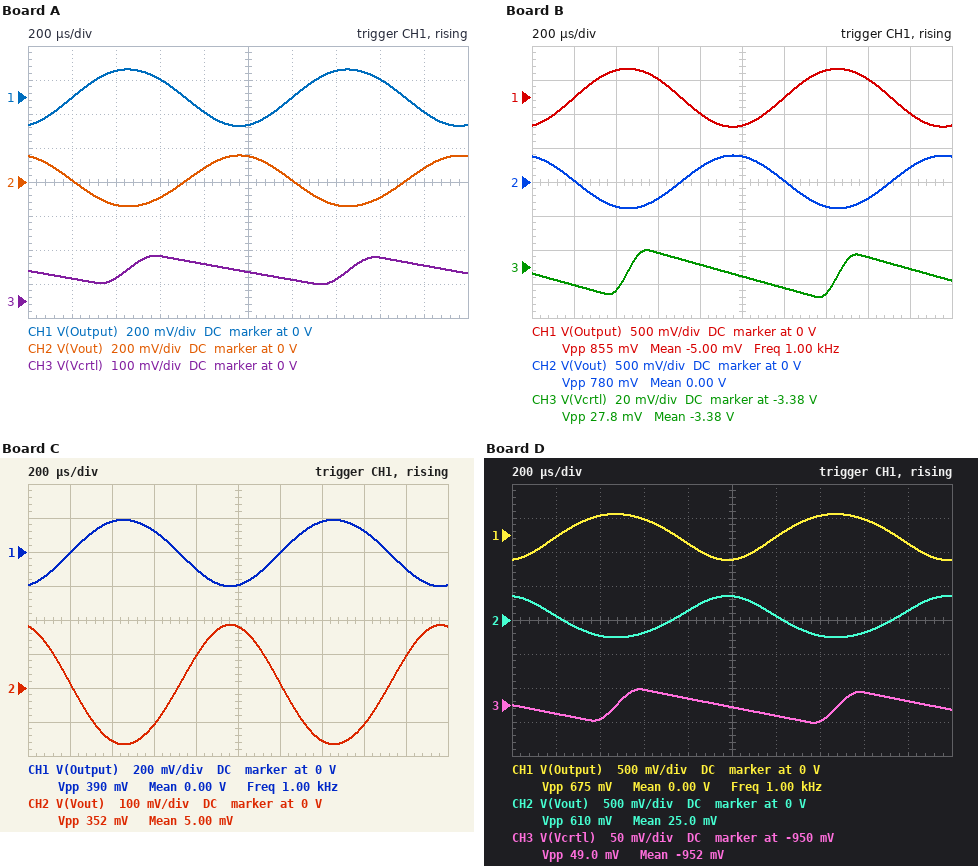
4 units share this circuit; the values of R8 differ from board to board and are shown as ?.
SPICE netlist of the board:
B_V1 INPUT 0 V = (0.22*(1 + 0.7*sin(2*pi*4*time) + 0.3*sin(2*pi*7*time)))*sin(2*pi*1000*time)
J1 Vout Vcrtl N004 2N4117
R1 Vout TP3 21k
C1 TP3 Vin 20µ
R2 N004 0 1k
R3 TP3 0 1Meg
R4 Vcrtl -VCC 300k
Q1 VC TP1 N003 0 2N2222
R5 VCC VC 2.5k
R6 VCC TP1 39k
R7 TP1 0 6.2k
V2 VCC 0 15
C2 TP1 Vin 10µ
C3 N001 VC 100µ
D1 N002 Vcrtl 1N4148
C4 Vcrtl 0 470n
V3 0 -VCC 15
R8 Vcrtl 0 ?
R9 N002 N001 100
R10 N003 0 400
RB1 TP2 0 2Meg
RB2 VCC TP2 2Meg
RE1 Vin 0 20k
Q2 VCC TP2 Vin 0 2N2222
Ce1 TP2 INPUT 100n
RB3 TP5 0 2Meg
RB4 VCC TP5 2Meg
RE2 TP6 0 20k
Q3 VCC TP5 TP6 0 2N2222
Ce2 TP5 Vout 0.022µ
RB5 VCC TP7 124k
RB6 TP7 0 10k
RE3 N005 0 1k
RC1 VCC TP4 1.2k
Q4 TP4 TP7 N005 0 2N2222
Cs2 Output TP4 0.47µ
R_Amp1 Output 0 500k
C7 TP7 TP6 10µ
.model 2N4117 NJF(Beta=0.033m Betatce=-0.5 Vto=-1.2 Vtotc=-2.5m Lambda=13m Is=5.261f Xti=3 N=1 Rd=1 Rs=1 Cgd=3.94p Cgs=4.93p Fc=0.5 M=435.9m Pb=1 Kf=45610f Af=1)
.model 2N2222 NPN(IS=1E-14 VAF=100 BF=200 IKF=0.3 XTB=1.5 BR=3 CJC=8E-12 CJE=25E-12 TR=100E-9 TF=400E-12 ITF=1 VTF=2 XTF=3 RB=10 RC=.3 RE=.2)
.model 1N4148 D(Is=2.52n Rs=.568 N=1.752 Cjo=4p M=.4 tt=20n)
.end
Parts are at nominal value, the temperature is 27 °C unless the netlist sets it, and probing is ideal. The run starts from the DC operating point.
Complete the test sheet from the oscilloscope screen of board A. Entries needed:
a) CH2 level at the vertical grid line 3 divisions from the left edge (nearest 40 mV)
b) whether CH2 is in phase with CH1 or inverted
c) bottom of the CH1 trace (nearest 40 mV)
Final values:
-80 mV
inverted
-160 mV
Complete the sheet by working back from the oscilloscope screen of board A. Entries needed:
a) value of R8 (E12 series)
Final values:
22 kΩ
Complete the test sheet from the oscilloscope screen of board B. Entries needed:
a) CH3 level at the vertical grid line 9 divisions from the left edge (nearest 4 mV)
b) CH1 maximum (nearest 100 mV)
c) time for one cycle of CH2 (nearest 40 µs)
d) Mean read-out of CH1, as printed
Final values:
-3.380 V
400 mV
1.00 ms
-5.00 mV
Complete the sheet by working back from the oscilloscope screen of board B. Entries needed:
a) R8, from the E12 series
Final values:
150 kΩ
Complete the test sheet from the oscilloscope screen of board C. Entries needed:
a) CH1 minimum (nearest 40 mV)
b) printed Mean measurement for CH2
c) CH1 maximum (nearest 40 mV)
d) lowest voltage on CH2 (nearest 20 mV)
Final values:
-200 mV
5.00 mV
200 mV
-160 mV
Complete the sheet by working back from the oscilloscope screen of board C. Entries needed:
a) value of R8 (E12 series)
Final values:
33 kΩ
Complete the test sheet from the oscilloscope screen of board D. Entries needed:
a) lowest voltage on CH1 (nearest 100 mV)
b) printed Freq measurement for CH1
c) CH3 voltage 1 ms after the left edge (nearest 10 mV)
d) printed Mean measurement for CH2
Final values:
-400 mV
1.00 kHz
-950 mV
25.0 mV
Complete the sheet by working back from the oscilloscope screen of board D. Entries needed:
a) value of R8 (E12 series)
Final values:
56 kΩ
